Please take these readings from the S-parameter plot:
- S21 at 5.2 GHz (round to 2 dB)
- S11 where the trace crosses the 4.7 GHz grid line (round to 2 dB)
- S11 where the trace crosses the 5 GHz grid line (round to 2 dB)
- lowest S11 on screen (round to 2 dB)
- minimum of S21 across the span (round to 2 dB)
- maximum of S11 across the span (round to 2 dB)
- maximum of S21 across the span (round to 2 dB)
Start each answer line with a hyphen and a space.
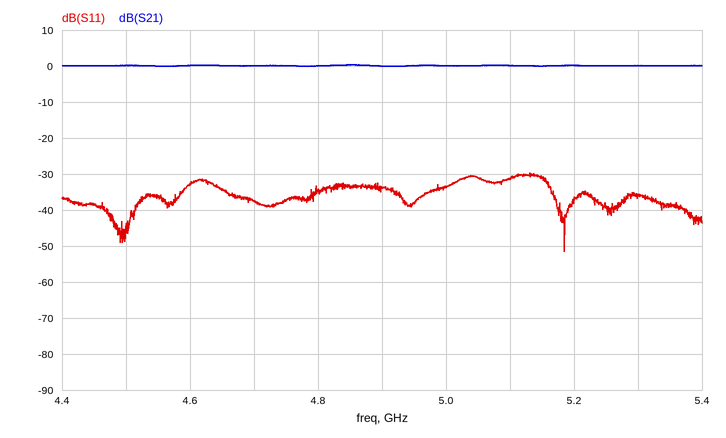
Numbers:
- 0 dB
- -38 dB
- -34 dB
- -52 dB
- 0 dB
- -30 dB
- 0 dB
